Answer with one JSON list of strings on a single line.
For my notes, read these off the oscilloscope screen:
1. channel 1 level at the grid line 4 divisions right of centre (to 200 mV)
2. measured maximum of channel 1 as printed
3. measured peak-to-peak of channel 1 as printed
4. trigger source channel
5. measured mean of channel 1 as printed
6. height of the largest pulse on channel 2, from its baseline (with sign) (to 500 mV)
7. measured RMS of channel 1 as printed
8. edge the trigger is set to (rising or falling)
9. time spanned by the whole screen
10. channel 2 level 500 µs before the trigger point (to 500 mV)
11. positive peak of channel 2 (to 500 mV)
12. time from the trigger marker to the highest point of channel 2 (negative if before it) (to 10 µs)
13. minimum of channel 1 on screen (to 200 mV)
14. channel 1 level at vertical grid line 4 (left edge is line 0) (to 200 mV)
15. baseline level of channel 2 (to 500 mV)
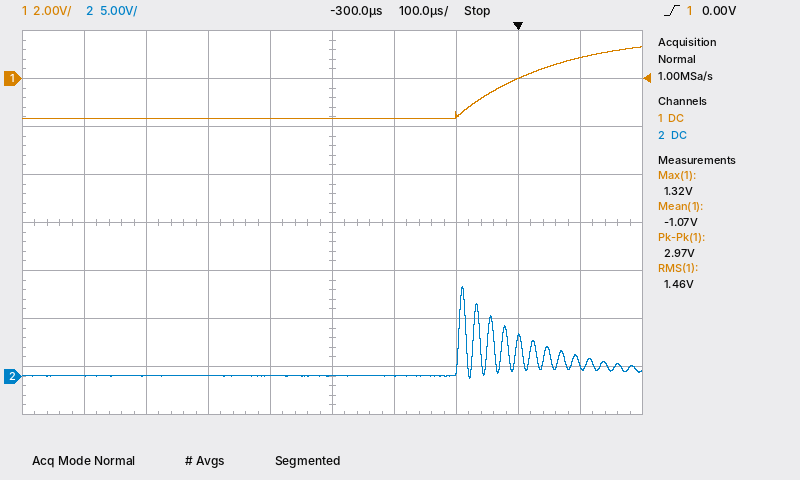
["800 mV", "1.32 V", "2.97 V", "channel 1", "-1.07 V", "+9.5 V", "1.46 V", "rising", "1 ms", "0.0 V", "9.5 V", "-90 µs", "-1.6 V", "-1.6 V", "0.0 V"]
